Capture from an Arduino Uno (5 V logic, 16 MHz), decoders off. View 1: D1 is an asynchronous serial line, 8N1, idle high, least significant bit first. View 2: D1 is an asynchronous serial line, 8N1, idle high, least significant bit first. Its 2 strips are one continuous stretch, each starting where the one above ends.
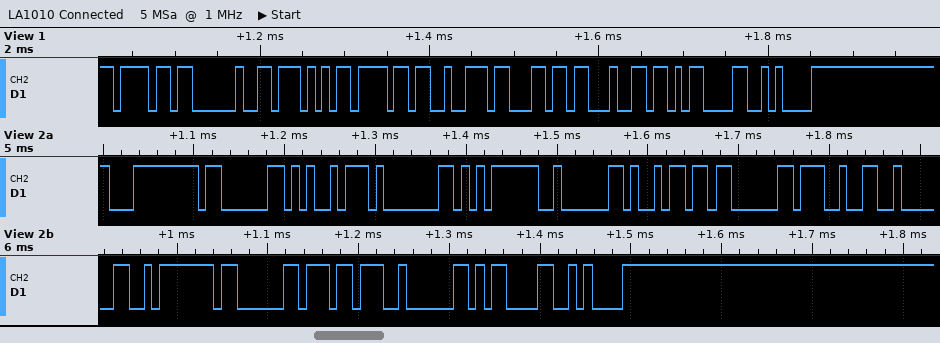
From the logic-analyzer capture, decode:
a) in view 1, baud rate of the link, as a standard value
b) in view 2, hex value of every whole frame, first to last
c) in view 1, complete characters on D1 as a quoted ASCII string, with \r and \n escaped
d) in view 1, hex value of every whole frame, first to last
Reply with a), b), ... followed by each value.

a) 115200 baud
b) FC 03 A5 01 F5 02 69 03 27 02 FA 03 B7 02 0D 0A
c) "o World\r\n"
d) 6F 20 57 6F 72 6C 64 0D 0A
